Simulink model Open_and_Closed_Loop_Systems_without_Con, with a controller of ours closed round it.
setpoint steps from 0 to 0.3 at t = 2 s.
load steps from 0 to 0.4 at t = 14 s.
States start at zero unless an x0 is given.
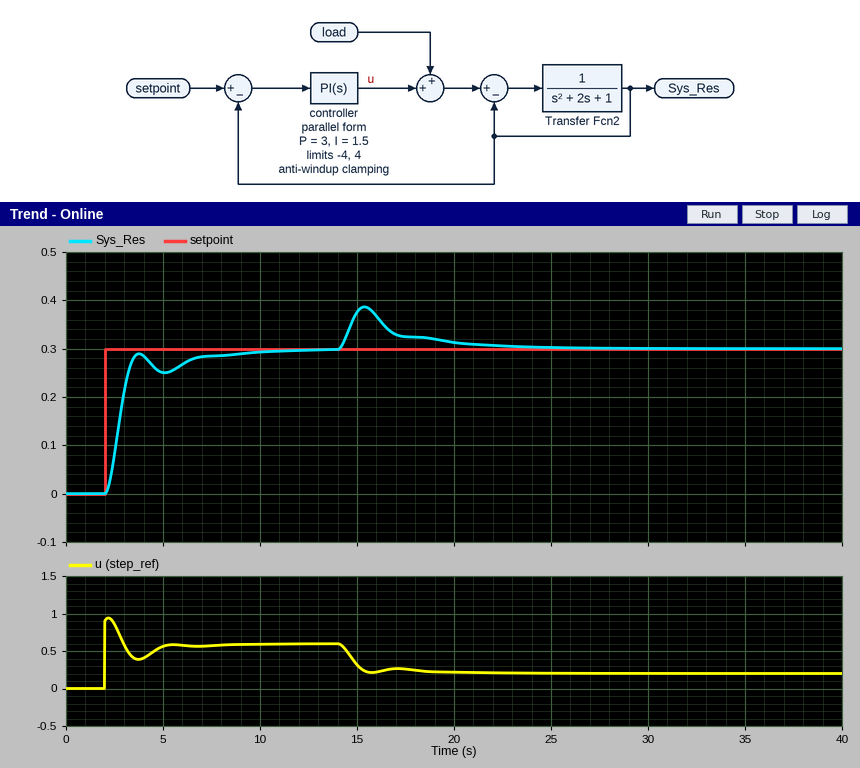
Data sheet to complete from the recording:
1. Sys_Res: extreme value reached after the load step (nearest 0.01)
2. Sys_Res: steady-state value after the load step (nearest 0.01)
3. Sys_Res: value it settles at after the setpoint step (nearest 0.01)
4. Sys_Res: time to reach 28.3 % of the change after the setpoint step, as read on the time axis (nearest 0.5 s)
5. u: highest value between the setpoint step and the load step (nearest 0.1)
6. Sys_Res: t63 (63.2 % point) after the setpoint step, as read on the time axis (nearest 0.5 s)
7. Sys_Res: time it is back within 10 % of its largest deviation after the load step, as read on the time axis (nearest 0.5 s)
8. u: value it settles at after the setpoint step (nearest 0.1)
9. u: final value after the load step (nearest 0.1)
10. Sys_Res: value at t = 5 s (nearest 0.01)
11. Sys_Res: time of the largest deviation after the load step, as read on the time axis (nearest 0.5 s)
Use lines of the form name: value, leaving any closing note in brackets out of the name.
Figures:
Sys_Res: extreme value reached after the load step: 0.39
Sys_Res: steady-state value after the load step: 0.30
Sys_Res: value it settles at after the setpoint step: 0.30
Sys_Res: time to reach 28.3 % of the change after the setpoint step, as read on the time axis: 2.5 s
u: highest value between the setpoint step and the load step: 0.9
Sys_Res: t63 (63.2 % point) after the setpoint step, as read on the time axis: 3.0 s
Sys_Res: time it is back within 10 % of its largest deviation after the load step, as read on the time axis: 21.0 s
u: value it settles at after the setpoint step: 0.6
u: final value after the load step: 0.2
Sys_Res: value at t = 5 s: 0.25
Sys_Res: time of the largest deviation after the load step, as read on the time axis: 15.5 s
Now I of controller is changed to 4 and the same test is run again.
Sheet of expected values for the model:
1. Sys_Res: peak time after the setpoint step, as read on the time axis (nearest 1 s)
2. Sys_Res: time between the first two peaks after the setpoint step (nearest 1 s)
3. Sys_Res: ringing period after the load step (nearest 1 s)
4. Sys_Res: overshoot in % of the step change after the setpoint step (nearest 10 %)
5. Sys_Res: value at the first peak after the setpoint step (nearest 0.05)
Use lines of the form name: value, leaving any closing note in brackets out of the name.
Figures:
Sys_Res: peak time after the setpoint step, as read on the time axis: 4 s
Sys_Res: time between the first two peaks after the setpoint step: 3 s
Sys_Res: ringing period after the load step: 3 s
Sys_Res: overshoot in % of the step change after the setpoint step: 30 %
Sys_Res: value at the first peak after the setpoint step: 0.40
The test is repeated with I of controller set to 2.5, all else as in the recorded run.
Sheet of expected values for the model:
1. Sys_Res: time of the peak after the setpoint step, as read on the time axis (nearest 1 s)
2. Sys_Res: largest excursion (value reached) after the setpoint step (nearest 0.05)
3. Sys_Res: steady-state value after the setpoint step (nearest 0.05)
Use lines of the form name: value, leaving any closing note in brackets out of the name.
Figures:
Sys_Res: time of the peak after the setpoint step, as read on the time axis: 4 s
Sys_Res: largest excursion (value reached) after the setpoint step: 0.35
Sys_Res: steady-state value after the setpoint step: 0.30
